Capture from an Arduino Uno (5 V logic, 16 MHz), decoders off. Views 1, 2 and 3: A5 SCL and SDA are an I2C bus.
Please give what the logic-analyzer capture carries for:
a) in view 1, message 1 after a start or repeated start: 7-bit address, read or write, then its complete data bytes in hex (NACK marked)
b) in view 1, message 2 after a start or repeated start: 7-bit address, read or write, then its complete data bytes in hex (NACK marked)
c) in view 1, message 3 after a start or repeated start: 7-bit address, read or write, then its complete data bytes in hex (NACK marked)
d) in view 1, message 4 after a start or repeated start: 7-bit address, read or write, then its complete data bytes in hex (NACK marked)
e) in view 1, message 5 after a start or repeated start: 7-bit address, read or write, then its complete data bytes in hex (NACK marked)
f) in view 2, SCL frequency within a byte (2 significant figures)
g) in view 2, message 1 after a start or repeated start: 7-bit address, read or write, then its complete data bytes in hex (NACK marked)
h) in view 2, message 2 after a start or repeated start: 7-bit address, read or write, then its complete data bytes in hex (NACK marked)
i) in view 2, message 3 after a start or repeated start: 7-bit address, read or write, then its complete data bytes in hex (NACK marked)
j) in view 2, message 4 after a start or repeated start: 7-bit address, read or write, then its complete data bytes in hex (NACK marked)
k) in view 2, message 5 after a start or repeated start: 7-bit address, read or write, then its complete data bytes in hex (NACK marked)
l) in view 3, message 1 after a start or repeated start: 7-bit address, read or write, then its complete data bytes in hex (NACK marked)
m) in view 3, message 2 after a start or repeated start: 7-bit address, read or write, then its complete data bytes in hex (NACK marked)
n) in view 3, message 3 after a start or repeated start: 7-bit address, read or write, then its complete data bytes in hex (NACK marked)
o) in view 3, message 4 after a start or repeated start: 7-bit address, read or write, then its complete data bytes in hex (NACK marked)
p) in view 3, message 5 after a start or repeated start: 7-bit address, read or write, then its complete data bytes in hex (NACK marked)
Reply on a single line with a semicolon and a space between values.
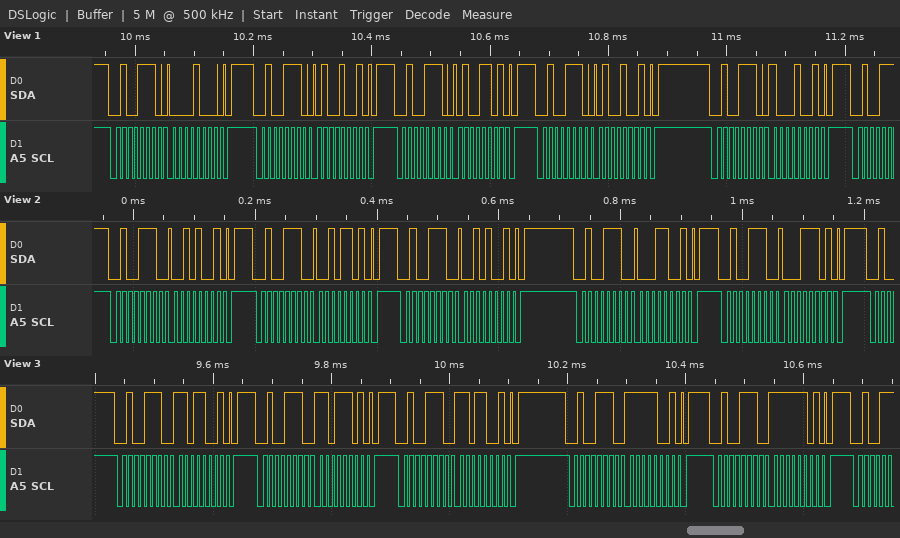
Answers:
0x27 write: 08; 0x27 write: 49; 0x27 write: 4D; 0x27 write: 49; 0x27 write: 89; 100 kHz; 0x27 write: 29; 0x27 write: 2D; 0x27 write: 29; 0x27 write: 19; 0x27 write: 1D; 0x27 write: D9; 0x27 write: DD; 0x27 write: D9; 0x27 write: F9; 0x27 write: FD
